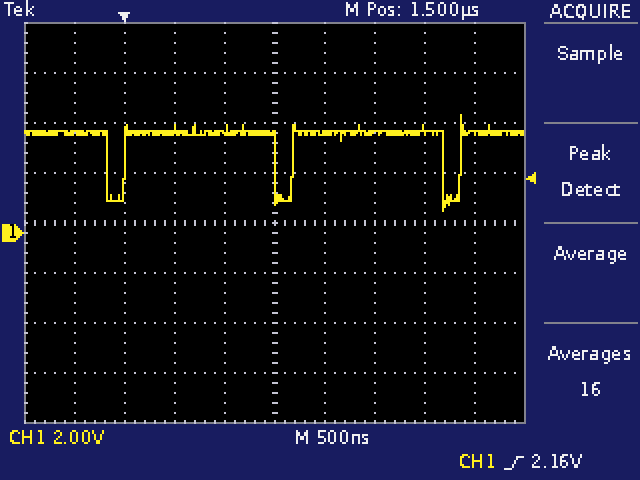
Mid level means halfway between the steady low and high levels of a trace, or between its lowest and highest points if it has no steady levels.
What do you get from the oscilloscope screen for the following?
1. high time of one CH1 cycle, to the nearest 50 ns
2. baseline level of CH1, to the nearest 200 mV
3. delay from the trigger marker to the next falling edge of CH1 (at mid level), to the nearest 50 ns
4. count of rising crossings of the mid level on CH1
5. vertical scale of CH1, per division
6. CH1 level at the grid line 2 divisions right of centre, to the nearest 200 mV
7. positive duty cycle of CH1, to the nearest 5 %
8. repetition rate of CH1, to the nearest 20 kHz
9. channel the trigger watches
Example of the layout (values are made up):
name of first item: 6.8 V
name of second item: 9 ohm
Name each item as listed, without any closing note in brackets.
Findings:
high time of one CH1 cycle, to the nearest 50 ns: 1.50 µs
baseline level of CH1, to the nearest 200 mV: 4.0 V
delay from the trigger marker to the next falling edge of CH1 (at mid level), to the nearest 50 ns: 1.50 µs
count of rising crossings of the mid level on CH1: 3
vertical scale of CH1, per division: 2 V
CH1 level at the grid line 2 divisions right of centre, to the nearest 200 mV: 4.0 V
positive duty cycle of CH1, to the nearest 5 %: 90 %
repetition rate of CH1, to the nearest 20 kHz: 600 kHz
channel the trigger watches: CH1
